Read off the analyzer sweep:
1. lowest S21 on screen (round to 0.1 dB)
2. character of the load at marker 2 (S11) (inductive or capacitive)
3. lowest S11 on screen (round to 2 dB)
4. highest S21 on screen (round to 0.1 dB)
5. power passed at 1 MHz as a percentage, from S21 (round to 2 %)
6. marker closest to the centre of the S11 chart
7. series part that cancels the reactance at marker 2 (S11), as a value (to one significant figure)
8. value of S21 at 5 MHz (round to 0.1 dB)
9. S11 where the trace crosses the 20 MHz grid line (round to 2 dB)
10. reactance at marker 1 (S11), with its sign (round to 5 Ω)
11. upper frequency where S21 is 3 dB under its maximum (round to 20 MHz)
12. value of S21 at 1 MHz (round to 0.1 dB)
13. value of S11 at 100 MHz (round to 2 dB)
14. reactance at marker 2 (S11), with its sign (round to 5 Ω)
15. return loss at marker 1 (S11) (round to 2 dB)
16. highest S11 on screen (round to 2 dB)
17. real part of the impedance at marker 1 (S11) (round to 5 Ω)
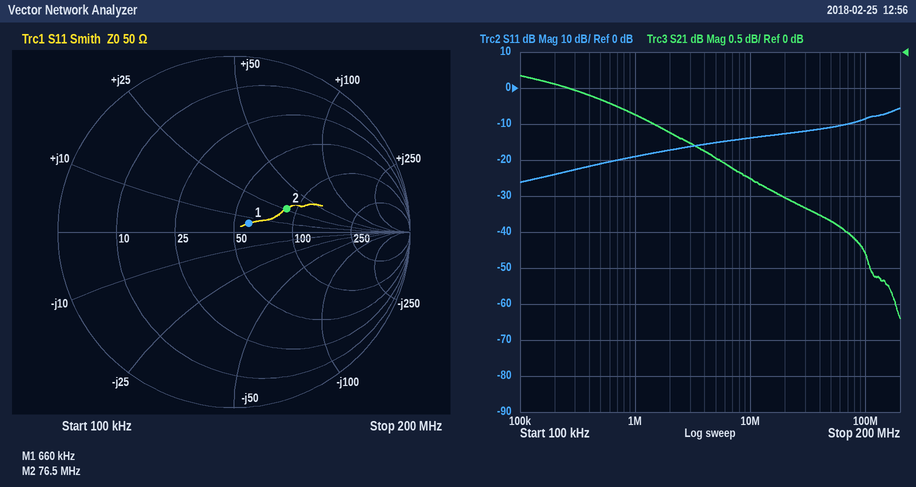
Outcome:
-3.7 dB
inductive
-26 dB
-0.3 dB
82 %
marker 1
80 pF
-1.5 dB
-12 dB
+5 Ω
160 MHz
-0.9 dB
-8 dB
+25 Ω
20 dB
-6 dB
60 Ω
